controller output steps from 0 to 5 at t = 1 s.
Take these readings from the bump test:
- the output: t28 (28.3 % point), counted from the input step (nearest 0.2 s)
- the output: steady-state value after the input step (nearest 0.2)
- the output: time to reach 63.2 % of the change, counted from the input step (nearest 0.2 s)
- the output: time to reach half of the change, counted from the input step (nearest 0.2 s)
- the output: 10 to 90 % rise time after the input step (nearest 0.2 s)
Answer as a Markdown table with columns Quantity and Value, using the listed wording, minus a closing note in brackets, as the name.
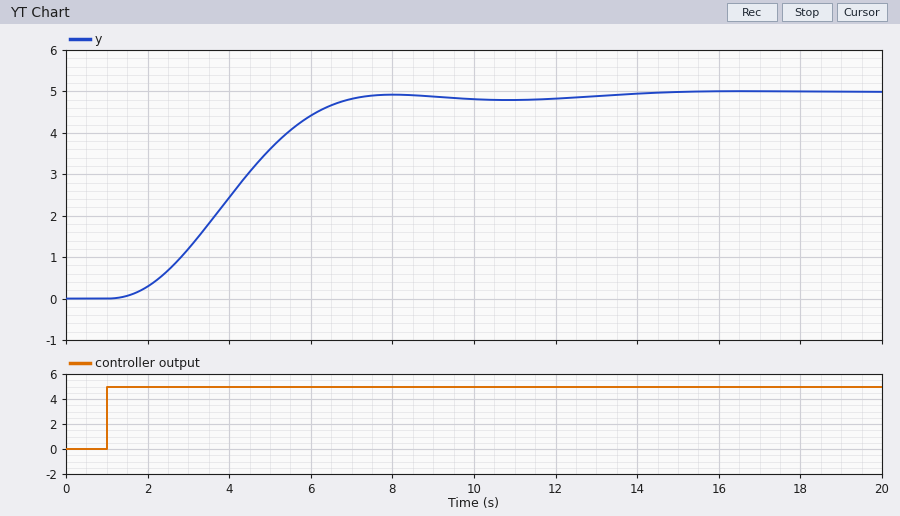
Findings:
| Quantity | Value |
|---|---|
| the output: t28 (28.3 % point), counted from the input step | 2.2 s |
| the output: steady-state value after the input step | 5.0 |
| the output: time to reach 63.2 % of the change, counted from the input step | 3.6 s |
| the output: time to reach half of the change, counted from the input step | 3.0 s |
| the output: 10 to 90 % rise time after the input step | 3.8 s |
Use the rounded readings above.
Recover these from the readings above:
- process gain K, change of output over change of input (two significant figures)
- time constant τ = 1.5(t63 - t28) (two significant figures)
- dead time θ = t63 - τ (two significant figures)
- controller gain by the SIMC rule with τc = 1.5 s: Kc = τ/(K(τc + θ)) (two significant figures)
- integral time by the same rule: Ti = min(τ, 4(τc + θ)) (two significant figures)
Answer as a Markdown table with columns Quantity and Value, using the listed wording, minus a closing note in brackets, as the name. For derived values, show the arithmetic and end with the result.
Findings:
| Quantity | Value |
|---|---|
| process gain K, change of output over change of input | (5 - 0) / 5 = 1.0 |
| time constant τ = 1.5(t63 - t28) | 1.5 × (3.6 - 2.2) = 2.1 s |
| dead time θ = t63 - τ | 3.6 - 2.1 = 1.5 s |
| controller gain by the SIMC rule with τc = 1.5 s: Kc = τ/(K(τc + θ)) | 2.1 / (1 × (1.5 + 1.5)) = 0.70 |
| integral time by the same rule: Ti = min(τ, 4(τc + θ)) | min(2.1, 4 × (1.5 + 1.5)) = 2.1 s |
